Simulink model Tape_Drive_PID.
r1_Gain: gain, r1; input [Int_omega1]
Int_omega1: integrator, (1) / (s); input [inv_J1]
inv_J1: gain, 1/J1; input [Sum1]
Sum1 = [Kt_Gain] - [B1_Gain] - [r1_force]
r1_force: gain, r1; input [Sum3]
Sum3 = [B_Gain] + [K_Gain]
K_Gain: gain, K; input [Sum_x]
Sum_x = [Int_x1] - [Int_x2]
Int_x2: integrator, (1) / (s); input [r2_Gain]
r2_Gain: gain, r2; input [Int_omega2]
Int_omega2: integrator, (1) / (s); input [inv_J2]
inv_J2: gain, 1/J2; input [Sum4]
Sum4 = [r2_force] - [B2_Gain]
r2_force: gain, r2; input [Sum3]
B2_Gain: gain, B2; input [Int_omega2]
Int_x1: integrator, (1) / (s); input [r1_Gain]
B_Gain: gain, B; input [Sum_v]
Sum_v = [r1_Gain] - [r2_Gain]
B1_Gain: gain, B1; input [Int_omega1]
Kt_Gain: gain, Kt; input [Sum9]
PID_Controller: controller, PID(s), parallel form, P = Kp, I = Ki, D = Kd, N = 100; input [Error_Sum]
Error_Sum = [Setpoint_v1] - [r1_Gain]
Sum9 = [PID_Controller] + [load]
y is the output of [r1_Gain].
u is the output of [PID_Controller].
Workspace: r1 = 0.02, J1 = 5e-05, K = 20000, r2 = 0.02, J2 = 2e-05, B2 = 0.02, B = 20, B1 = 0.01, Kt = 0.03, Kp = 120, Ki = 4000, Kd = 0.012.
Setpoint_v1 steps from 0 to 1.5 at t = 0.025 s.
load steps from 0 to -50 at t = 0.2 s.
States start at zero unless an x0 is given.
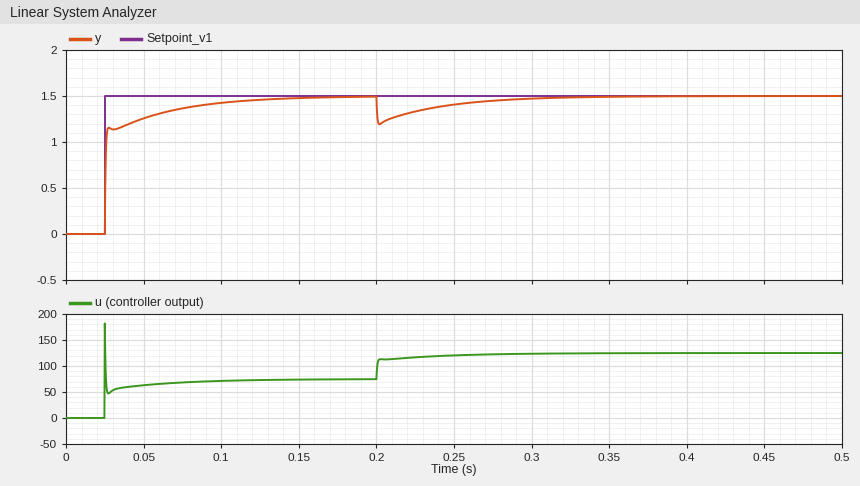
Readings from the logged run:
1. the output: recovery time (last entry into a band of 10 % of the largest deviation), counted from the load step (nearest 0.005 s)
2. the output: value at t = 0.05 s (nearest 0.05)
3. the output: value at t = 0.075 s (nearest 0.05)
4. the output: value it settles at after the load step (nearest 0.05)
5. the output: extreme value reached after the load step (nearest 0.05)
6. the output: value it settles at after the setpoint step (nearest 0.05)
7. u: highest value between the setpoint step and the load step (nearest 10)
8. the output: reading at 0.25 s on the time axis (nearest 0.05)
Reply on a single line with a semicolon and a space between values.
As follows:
0.100 s; 1.25; 1.35; 1.50; 1.20; 1.50; 180; 1.40
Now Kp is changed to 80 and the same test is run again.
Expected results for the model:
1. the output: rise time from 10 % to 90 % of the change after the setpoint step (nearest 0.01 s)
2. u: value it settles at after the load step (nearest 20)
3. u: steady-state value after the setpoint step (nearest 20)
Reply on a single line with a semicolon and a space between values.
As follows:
0.04 s; 120; 80
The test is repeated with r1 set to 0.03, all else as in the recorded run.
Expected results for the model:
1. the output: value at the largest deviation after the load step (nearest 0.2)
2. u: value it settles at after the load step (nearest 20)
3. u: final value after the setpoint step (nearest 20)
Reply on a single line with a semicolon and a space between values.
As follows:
1.2; 140; 100
